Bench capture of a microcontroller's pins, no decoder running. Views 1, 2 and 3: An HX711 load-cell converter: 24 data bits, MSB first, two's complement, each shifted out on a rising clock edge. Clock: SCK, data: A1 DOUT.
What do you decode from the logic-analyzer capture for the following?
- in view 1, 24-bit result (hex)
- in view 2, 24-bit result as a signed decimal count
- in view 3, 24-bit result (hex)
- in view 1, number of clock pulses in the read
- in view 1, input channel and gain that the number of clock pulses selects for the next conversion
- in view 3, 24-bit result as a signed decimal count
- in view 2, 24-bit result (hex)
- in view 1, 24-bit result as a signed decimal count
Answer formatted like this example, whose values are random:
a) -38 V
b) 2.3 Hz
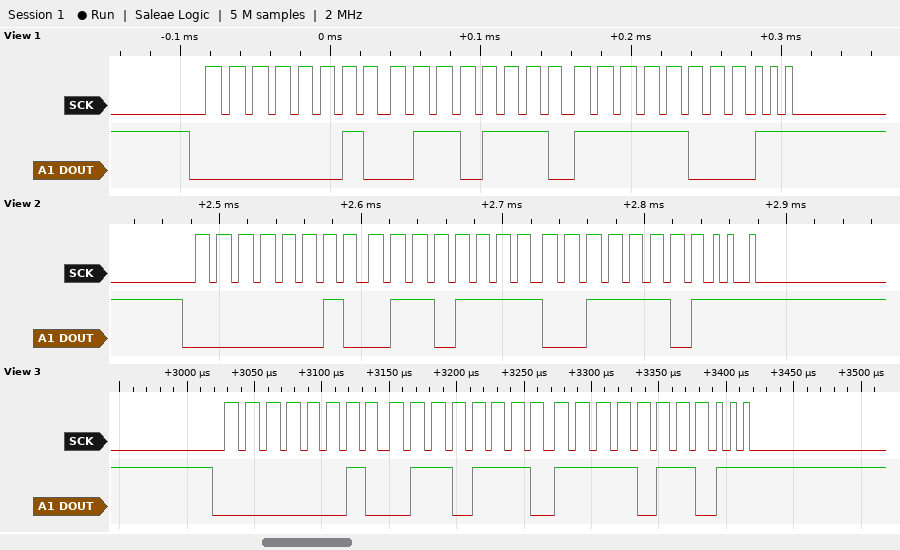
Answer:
a) 0x026EF8
b) 159549
c) 0x026EF6
d) 27
e) channel A, gain 64
f) 159478
g) 0x026F3D
h) 159480
